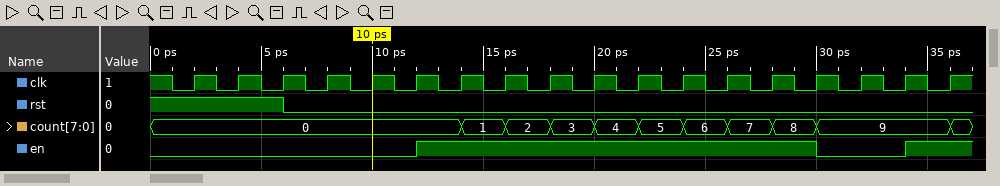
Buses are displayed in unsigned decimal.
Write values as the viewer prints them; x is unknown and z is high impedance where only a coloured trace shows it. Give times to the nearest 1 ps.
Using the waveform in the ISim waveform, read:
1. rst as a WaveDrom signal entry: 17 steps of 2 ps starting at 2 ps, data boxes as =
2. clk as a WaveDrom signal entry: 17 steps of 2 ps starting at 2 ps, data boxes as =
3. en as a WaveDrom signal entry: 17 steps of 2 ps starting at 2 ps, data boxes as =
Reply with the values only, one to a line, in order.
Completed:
{name: 'rst', wave: '1.0..............'}
{name: 'clk', wave: 'p................'}
{name: 'en', wave: '0....1........0.1'}
